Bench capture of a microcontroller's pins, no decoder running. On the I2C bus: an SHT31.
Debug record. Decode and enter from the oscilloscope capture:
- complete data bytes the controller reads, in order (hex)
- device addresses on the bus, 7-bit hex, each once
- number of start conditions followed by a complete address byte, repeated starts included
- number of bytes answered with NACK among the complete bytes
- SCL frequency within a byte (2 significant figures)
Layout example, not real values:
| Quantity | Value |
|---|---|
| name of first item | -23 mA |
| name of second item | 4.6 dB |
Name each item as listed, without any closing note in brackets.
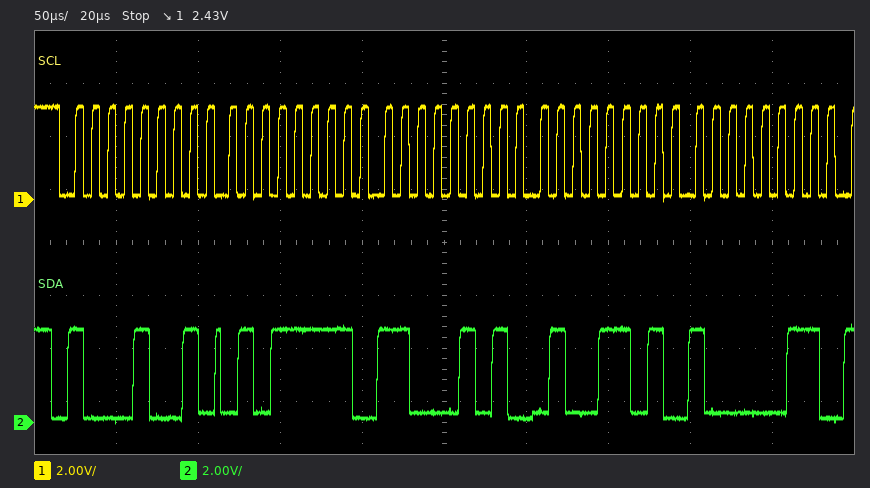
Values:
| Quantity | Value |
|---|---|
| complete data bytes the controller reads, in order | 5F C5 4D 83 |
| device addresses on the bus, 7-bit hex, each once | 0x44 |
| number of start conditions followed by a complete address byte, repeated starts included | 1 |
| number of bytes answered with NACK among the complete bytes | 0 |
| SCL frequency within a byte | 100 kHz |
